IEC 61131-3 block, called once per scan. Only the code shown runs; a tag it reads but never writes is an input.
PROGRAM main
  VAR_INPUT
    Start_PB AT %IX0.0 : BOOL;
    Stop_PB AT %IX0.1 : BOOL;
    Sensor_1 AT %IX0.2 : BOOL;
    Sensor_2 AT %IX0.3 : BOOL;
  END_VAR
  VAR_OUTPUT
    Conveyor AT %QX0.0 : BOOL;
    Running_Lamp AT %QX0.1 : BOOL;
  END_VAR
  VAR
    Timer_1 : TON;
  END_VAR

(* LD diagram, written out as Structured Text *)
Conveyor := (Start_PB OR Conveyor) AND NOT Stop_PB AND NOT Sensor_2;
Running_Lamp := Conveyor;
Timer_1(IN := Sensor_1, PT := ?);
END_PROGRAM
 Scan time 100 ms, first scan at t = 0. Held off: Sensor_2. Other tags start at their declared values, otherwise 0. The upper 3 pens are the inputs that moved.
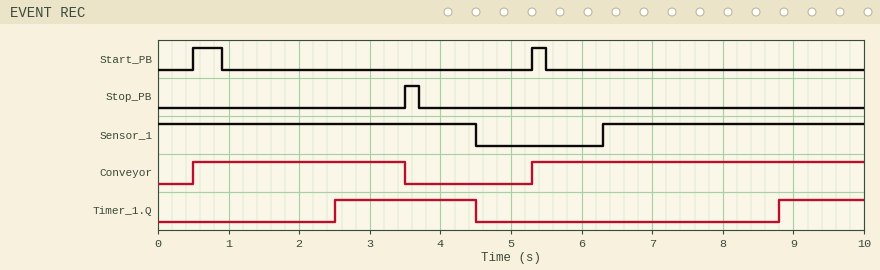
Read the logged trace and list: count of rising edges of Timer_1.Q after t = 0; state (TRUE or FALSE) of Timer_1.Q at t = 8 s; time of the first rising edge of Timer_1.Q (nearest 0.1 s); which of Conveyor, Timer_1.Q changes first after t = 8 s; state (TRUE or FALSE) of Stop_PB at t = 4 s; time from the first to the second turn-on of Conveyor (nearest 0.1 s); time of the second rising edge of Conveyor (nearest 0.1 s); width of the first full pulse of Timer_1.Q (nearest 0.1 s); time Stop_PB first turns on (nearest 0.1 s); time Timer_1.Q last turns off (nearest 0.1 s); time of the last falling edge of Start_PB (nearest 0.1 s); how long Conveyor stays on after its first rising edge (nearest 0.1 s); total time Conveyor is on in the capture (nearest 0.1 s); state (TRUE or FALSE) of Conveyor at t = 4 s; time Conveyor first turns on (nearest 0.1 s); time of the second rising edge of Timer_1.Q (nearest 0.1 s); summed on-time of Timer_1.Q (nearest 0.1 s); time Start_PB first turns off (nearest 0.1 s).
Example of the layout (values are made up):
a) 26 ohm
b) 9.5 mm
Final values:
a) 2
b) FALSE
c) 2.5 s
d) Timer_1.Q
e) FALSE
f) 4.8 s
g) 5.3 s
h) 2.0 s
i) 3.5 s
j) 4.5 s
k) 5.5 s
l) 3.0 s
m) 7.7 s
n) FALSE
o) 0.5 s
p) 8.8 s
q) 3.2 s
r) 0.9 s
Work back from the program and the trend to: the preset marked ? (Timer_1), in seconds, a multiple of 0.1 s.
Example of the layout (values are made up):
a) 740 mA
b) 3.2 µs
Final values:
a) 2.5 s
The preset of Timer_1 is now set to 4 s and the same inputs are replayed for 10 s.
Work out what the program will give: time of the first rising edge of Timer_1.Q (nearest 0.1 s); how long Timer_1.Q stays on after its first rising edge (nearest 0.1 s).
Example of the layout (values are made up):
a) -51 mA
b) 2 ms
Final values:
a) 4.0 s
b) 0.5 s
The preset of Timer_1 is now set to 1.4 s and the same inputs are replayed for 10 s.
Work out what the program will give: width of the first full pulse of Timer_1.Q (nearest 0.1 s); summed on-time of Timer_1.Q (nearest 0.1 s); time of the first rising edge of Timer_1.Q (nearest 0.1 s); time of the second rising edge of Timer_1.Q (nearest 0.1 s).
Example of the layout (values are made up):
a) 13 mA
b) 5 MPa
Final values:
a) 3.1 s
b) 5.4 s
c) 1.4 s
d) 7.7 s
